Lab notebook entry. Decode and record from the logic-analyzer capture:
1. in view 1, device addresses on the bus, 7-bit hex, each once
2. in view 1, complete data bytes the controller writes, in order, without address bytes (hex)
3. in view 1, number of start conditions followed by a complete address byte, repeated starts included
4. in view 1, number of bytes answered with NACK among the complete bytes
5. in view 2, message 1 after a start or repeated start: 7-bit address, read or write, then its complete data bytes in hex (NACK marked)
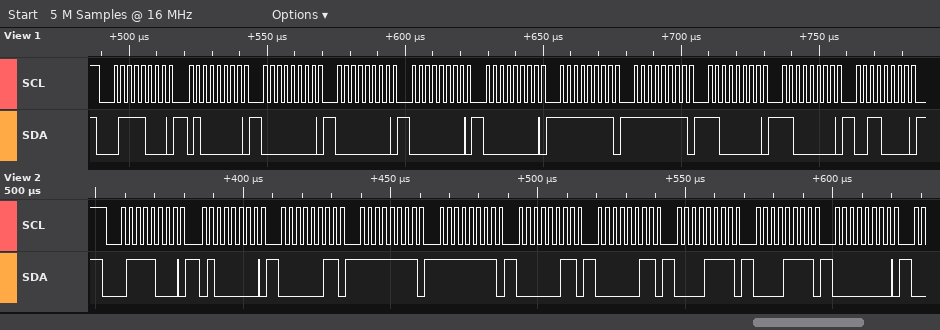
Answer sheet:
0x3C
40 00 00 00 00 FF FF C0 C0 30
1
0
0x3C write: 40 03 FF FF 03 03 0F 0F 00
